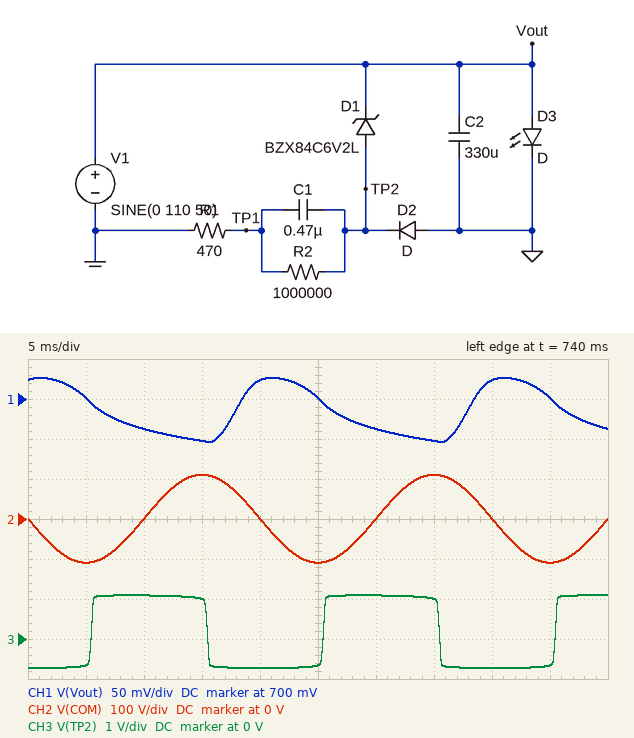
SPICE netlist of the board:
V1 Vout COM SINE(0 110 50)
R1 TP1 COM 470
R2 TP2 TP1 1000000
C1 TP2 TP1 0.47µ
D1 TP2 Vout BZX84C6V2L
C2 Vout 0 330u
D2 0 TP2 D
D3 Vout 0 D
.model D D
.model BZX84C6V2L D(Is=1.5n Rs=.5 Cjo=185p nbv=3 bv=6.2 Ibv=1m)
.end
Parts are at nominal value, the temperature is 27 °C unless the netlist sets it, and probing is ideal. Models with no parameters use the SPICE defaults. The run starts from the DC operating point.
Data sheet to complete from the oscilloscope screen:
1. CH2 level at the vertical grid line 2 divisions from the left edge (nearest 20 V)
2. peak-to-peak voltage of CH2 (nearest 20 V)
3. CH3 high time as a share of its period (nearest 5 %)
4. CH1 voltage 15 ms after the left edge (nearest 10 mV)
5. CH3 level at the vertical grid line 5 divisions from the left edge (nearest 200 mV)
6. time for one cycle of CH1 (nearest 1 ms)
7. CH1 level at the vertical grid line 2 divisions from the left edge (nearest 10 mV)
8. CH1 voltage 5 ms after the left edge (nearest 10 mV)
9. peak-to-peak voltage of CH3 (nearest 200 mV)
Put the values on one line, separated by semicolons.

0 V; 220 V; 50 %; 650 mV; -600 mV; 20 ms; 660 mV; 700 mV; 1.8 V
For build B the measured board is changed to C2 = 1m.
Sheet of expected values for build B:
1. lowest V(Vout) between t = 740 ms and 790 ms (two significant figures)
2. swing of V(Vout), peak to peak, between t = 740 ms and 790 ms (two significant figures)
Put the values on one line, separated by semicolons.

670 mV; 47 mV
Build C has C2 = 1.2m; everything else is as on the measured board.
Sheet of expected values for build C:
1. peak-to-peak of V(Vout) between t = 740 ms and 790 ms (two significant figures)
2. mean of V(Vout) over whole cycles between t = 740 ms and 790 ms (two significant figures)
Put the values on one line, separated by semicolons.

41 mV; 690 mV
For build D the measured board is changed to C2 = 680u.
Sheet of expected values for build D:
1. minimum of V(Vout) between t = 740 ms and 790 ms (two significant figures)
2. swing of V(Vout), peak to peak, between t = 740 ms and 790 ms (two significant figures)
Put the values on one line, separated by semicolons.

660 mV; 59 mV
